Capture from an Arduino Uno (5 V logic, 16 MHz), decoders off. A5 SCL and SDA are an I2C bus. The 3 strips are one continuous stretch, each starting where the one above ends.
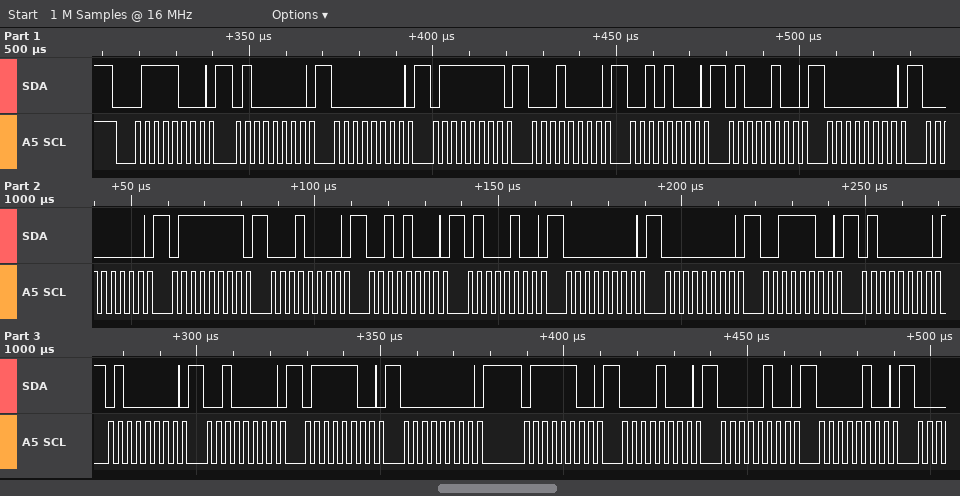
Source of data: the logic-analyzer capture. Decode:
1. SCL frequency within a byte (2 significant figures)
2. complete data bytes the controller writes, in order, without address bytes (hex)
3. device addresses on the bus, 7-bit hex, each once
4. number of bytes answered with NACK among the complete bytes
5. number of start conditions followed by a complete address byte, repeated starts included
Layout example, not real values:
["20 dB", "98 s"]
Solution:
["400 kHz", "40 00 7F 10 28 44 00 00 7F 10 28 44 00 00 3C 40 40 20 7C 00 7C 08 04 04", "0x3C", "0", "1"]
